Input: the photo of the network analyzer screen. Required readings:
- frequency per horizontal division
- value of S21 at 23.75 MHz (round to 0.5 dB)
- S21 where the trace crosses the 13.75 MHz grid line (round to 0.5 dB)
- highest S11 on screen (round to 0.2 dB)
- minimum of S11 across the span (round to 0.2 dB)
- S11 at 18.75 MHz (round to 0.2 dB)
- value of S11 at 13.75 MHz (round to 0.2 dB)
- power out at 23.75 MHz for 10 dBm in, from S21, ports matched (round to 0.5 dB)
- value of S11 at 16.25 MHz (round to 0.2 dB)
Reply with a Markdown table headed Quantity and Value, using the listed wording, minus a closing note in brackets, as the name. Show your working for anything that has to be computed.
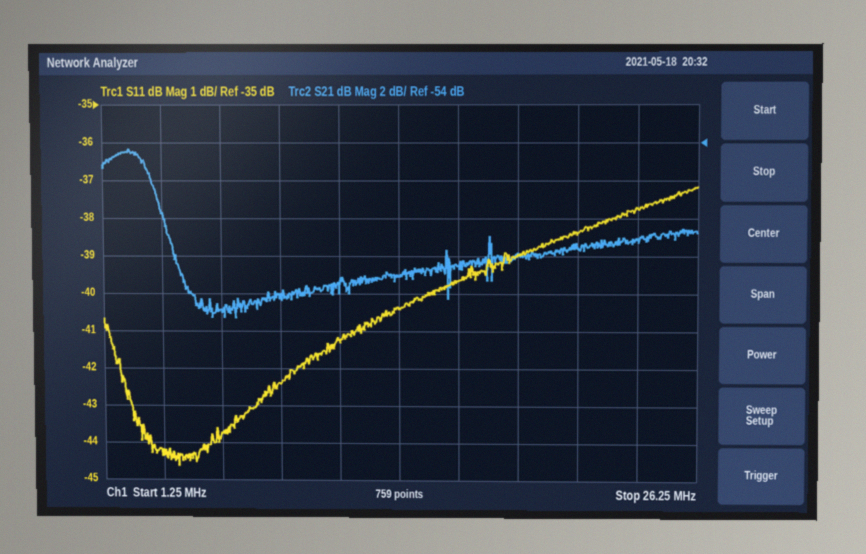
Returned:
| Quantity | Value |
|---|---|
| frequency per horizontal division | 2.5 MHz |
| value of S21 at 23.75 MHz | -59.0 dB |
| S21 where the trace crosses the 13.75 MHz grid line | -61.0 dB |
| highest S11 on screen | -37.2 dB |
| minimum of S11 across the span | -44.6 dB |
| S11 at 18.75 MHz | -39.0 dB |
| value of S11 at 13.75 MHz | -40.4 dB |
| power out at 23.75 MHz for 10 dBm in, from S21, ports matched | 10 dBm + (-59.0 dB) = -49.0 dBm |
| value of S11 at 16.25 MHz | -39.6 dB |
